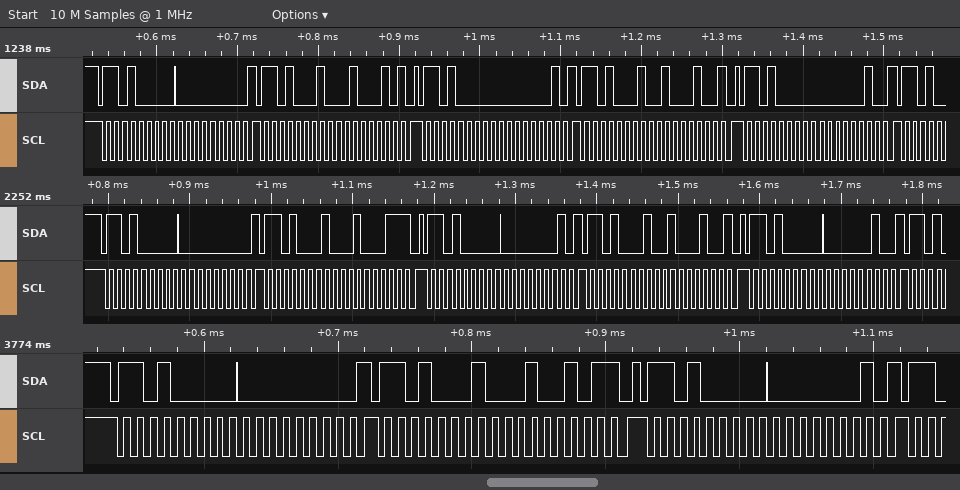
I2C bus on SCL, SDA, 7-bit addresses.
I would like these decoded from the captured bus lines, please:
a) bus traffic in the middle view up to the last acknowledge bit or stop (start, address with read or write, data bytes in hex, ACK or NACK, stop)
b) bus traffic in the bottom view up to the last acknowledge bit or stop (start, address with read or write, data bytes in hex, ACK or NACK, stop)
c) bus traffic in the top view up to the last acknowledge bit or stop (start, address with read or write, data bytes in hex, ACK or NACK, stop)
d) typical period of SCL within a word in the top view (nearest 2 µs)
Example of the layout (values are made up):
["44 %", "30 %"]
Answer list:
["start, address 68 write ACK, 00 ACK, repeated start, address 68 read ACK, 23 NACK, stop, start, address 68 write ACK, 01 ACK, repeated start, address 68 read ACK, 44 NACK, stop, start, address 68 write ACK, 02 ACK", "start, address 68 write ACK, 00 ACK, repeated start, address 68 read ACK, 25 NACK, stop, start, address 68 write ACK, 01 ACK", "start, address 68 write ACK, 00 ACK, repeated start, address 68 read ACK, 22 NACK, stop, start, address 68 write ACK, 01 ACK, repeated start, address 68 read ACK, 44 NACK, stop, start, address 68 write ACK, 02 ACK", "10 µs"]
